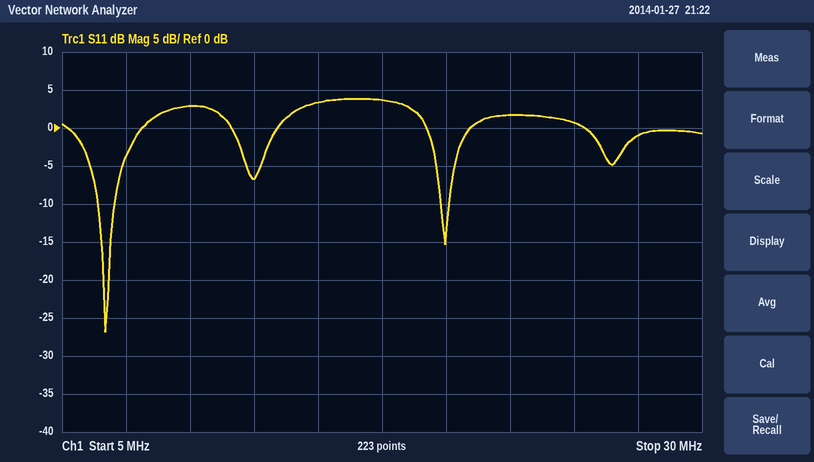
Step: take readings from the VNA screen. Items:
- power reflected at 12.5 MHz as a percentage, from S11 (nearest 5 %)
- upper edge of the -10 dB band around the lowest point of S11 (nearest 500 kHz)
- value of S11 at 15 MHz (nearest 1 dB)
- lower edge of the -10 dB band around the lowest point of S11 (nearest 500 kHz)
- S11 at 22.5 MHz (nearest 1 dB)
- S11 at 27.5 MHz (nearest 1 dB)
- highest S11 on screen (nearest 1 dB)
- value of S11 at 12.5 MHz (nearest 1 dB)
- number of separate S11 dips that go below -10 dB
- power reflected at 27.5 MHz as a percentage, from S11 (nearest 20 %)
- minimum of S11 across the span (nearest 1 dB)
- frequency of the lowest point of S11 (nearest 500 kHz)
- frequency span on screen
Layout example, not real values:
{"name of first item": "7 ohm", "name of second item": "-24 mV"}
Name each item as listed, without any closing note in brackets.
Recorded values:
{"power reflected at 12.5 MHz as a percentage, from S11": "20 %", "upper edge of the -10 dB band around the lowest point of S11": "7.0 MHz", "value of S11 at 15 MHz": "3 dB", "lower edge of the -10 dB band around the lowest point of S11": "6.5 MHz", "S11 at 22.5 MHz": "2 dB", "S11 at 27.5 MHz": "-1 dB", "highest S11 on screen": "4 dB", "value of S11 at 12.5 MHz": "-7 dB", "number of separate S11 dips that go below -10 dB": "2", "power reflected at 27.5 MHz as a percentage, from S11": "80 %", "minimum of S11 across the span": "-27 dB", "frequency of the lowest point of S11": "6.5 MHz", "frequency span on screen": "25 MHz"}
